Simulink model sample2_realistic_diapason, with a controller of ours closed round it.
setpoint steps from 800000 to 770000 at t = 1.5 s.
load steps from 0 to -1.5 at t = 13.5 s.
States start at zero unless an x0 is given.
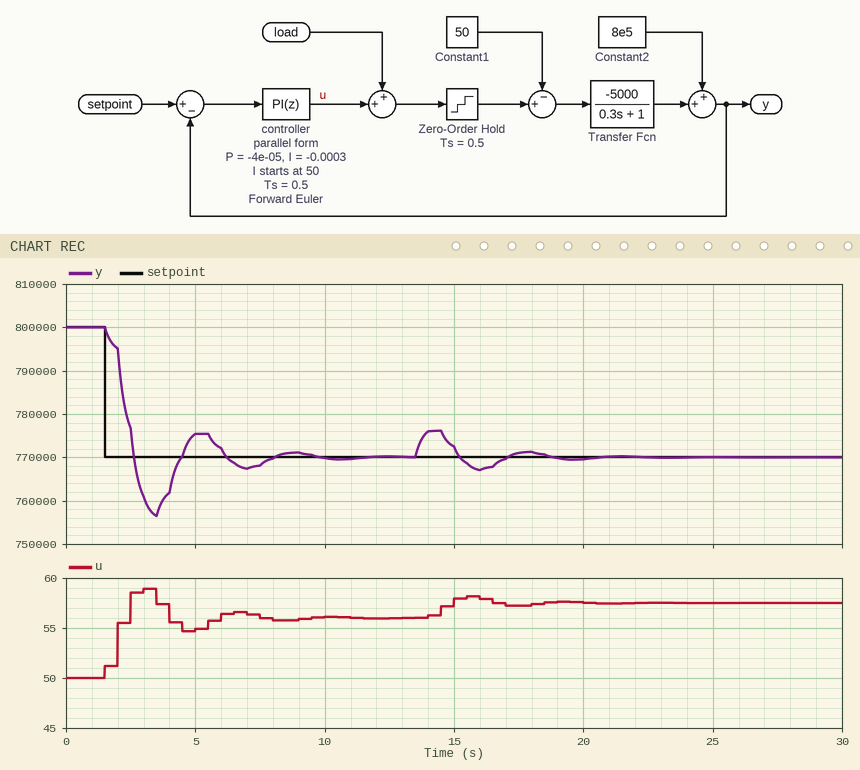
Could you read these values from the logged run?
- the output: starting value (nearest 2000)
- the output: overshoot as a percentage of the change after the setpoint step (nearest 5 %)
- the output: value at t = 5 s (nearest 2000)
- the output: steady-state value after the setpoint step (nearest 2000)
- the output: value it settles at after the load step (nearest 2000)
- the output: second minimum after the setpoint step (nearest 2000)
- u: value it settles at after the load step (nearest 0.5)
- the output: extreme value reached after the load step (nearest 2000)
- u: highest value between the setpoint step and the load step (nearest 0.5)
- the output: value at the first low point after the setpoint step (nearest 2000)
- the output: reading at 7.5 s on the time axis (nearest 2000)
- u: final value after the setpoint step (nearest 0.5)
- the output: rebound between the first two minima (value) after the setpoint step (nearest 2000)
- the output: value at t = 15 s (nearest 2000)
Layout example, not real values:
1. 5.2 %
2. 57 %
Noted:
1. 800000
2. 45 %
3. 776000
4. 770000
5. 770000
6. 768000
7. 57.5
8. 776000
9. 59.0
10. 756000
11. 768000
12. 56.0
13. 776000
14. 772000
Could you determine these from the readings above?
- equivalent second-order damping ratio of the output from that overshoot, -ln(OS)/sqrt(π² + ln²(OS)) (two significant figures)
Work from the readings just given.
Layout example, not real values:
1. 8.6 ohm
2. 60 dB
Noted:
1. 0.25
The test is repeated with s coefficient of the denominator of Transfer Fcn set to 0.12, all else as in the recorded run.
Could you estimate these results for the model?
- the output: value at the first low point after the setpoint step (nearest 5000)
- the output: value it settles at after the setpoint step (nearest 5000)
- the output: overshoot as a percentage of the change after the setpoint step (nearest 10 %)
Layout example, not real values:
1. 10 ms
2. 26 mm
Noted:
1. 760000
2. 770000
3. 40 %
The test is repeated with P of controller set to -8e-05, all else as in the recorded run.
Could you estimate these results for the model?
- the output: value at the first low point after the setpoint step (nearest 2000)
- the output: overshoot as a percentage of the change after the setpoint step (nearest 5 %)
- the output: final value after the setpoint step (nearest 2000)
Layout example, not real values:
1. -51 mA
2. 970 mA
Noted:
1. 762000
2. 25 %
3. 770000
